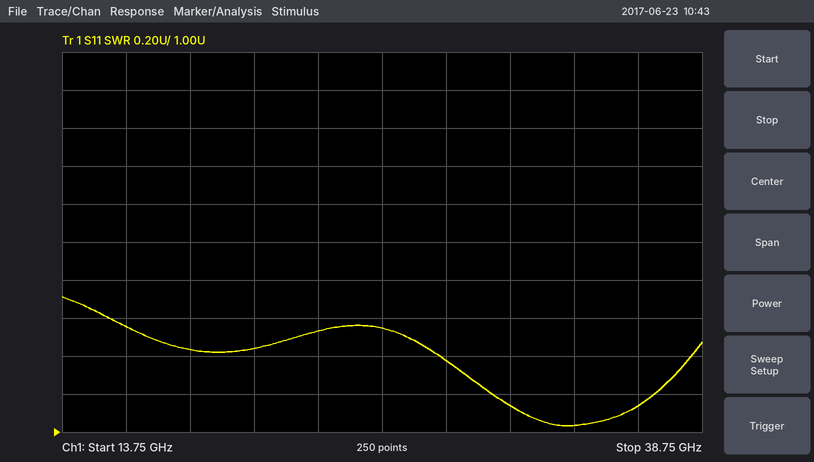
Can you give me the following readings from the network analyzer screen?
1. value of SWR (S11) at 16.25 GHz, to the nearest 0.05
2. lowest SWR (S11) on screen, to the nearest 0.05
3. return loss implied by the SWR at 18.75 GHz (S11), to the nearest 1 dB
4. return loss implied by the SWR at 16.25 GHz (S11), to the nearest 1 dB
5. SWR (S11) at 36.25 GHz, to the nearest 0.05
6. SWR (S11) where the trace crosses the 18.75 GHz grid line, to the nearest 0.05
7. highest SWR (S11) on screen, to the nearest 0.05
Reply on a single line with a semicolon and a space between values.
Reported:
1.55; 1.05; 15 dB; 13 dB; 1.15; 1.45; 1.70
